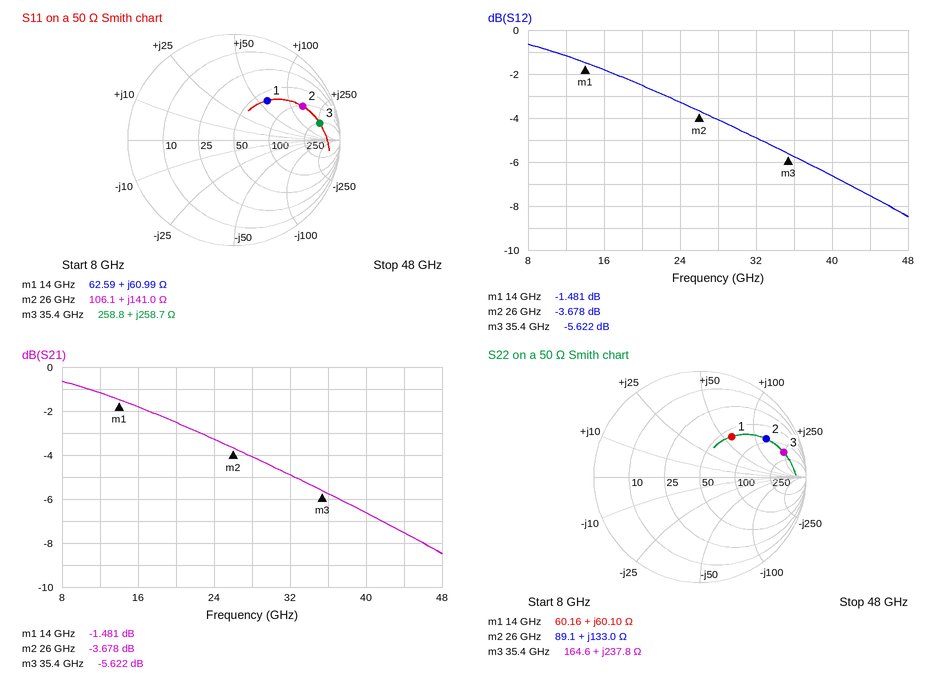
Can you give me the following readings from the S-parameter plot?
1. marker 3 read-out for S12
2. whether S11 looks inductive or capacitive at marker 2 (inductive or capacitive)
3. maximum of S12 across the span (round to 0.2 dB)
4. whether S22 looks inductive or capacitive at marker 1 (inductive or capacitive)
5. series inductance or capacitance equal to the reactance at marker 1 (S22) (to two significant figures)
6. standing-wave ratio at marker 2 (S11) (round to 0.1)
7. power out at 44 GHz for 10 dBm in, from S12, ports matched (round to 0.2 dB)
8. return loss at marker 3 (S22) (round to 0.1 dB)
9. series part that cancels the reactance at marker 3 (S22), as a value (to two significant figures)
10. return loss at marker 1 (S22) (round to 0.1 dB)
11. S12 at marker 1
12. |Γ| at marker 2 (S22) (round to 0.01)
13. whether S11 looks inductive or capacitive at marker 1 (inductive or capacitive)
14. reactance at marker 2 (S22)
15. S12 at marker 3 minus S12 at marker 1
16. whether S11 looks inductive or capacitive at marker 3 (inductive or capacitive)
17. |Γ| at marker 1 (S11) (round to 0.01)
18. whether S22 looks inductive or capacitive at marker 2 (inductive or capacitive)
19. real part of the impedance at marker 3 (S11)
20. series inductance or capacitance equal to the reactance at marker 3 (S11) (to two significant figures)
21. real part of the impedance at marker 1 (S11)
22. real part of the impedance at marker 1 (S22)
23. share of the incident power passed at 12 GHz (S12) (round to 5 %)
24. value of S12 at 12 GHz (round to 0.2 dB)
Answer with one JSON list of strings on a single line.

["-5.622 dB", "inductive", "-0.6 dB", "inductive", "680 pH", "6.2", "2.4 dBm", "1.7 dB", "19 fF", "6.3 dB", "-1.481 dB", "0.72", "inductive", "+133.0 Ω", "-4.141 dB", "inductive", "0.49", "inductive", "258.8 Ω", "1.2 nH", "62.59 Ω", "60.16 Ω", "75 %", "-1.2 dB"]
